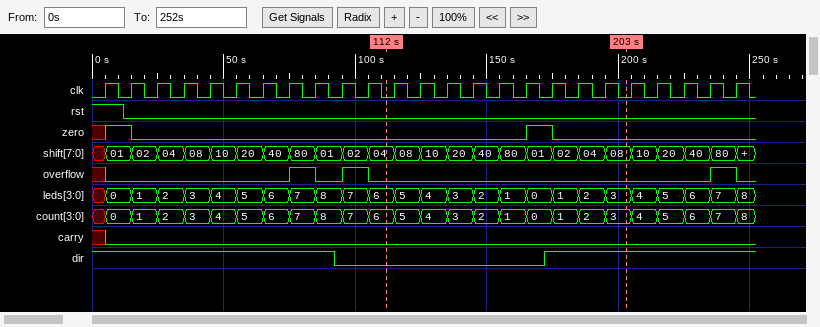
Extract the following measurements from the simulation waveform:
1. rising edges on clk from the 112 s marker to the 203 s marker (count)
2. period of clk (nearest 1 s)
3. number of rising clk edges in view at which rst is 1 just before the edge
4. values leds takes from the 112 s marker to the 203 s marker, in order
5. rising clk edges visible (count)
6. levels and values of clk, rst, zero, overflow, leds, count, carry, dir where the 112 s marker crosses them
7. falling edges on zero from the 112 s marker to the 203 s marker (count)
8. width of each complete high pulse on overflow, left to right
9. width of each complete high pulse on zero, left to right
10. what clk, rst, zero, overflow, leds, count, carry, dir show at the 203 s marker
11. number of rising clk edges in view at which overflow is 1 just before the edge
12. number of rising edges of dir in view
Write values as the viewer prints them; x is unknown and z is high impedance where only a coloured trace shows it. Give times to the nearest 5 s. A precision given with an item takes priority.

9
10 s
1
6, 5, 4, 3, 2, 1, 0, 1, 2, 3
25
clk=0, rst=0, zero=0, overflow=0, leds=6, count=6, carry=0, dir=0
1
10 s, 10 s, 10 s
10 s
clk=0, rst=0, zero=0, overflow=0, leds=3, count=3, carry=0, dir=1
3
1
